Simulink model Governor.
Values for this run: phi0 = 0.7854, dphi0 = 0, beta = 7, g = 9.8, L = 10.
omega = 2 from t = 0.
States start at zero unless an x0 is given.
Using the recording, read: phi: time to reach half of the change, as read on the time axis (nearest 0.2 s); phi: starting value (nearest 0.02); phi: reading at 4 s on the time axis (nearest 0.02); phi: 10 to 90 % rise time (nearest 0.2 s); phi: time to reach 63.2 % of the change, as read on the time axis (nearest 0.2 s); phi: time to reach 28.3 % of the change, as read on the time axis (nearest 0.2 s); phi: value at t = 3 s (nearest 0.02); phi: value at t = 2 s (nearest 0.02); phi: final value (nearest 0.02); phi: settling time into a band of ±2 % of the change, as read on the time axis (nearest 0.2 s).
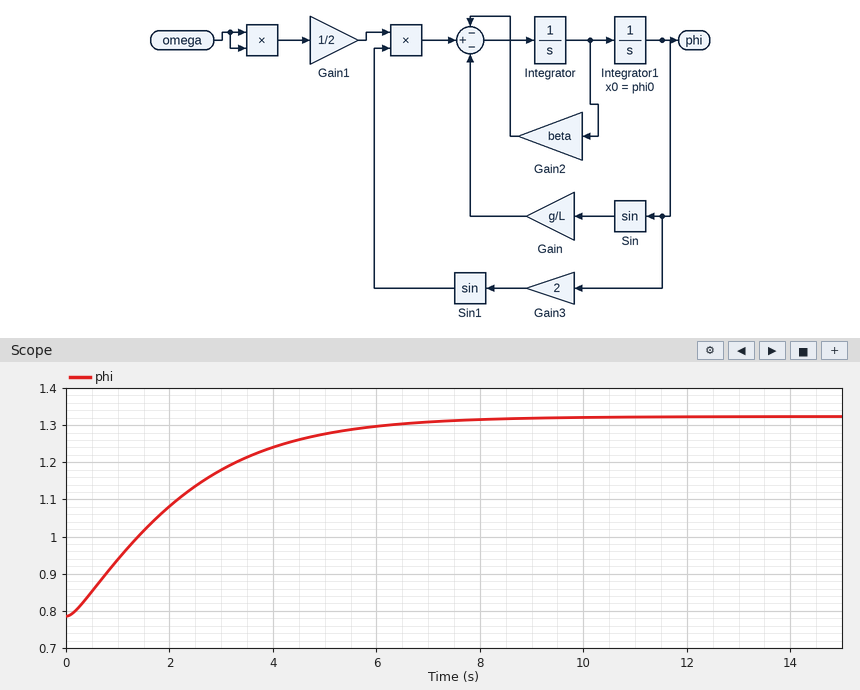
1.8 s
0.78
1.24
4.4 s
2.4 s
1.0 s
1.18
1.08
1.32
7.6 s
